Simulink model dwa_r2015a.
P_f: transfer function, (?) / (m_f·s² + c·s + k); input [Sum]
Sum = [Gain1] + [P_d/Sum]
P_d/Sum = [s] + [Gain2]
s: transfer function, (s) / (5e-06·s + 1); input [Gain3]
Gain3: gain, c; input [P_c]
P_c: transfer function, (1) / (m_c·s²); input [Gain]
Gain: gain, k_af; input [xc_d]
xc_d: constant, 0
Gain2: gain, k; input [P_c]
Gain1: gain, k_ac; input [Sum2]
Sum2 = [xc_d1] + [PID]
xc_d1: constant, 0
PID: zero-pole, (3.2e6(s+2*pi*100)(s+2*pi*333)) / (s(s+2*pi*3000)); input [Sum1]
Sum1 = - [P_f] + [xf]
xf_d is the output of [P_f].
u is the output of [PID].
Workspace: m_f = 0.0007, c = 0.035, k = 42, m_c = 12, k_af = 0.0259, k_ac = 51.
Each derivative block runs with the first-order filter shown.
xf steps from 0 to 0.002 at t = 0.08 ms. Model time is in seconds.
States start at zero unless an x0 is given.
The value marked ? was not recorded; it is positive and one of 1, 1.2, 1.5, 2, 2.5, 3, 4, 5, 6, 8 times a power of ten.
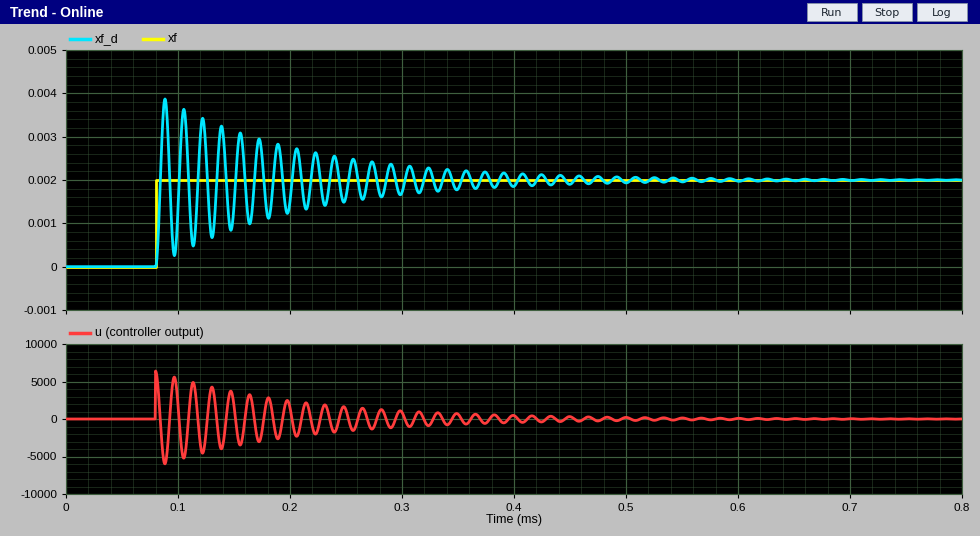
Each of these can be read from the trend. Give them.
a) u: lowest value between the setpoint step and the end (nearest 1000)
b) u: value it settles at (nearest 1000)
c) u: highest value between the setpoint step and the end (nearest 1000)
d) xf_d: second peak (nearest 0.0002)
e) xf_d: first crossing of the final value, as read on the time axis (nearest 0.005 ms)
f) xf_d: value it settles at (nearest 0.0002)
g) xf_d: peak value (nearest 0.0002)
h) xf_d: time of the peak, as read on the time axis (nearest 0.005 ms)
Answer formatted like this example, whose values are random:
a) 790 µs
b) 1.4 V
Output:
a) -6000
b) 0
c) 6000
d) 0.0036
e) 0.085 ms
f) 0.0020
g) 0.0038
h) 0.090 ms
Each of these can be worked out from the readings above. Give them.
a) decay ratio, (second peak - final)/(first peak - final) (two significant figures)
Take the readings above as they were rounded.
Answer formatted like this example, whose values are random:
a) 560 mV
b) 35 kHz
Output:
a) 0.89
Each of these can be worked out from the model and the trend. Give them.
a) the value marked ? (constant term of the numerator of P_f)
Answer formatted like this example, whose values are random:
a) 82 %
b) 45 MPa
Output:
a) 0.6
